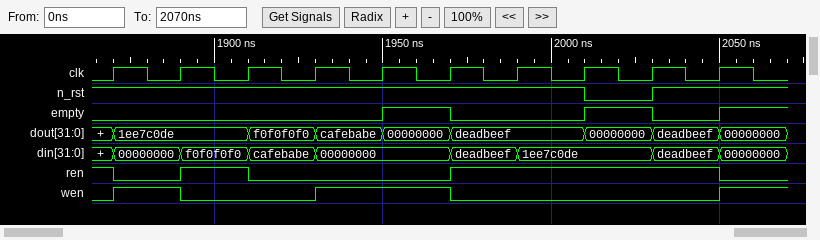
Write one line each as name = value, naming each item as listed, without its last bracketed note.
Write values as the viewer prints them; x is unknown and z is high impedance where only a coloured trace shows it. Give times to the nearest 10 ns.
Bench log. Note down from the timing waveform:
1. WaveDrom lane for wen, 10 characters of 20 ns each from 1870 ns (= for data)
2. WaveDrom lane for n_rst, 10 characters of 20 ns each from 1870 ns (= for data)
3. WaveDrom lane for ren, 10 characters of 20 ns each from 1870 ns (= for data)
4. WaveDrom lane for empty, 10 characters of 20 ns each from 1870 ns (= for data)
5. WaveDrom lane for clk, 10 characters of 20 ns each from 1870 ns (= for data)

WaveDrom lane for wen, 10 characters of 20 ns each from 1870 ns = {name: 'wen', wave: '10.1.0...1'}
WaveDrom lane for n_rst, 10 characters of 20 ns each from 1870 ns = {name: 'n_rst', wave: '1......01.'}
WaveDrom lane for ren, 10 characters of 20 ns each from 1870 ns = {name: 'ren', wave: '010..1...0'}
WaveDrom lane for empty, 10 characters of 20 ns each from 1870 ns = {name: 'empty', wave: '0...10.101'}
WaveDrom lane for clk, 10 characters of 20 ns each from 1870 ns = {name: 'clk', wave: 'p.........'}
